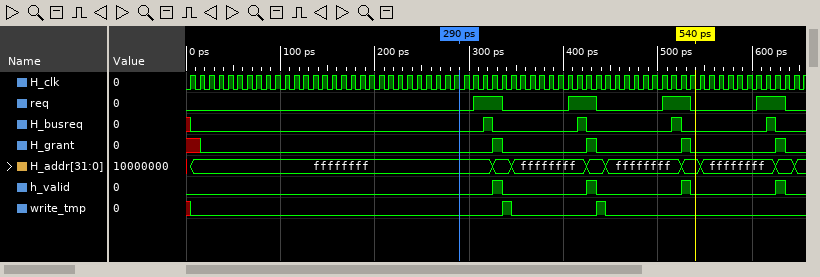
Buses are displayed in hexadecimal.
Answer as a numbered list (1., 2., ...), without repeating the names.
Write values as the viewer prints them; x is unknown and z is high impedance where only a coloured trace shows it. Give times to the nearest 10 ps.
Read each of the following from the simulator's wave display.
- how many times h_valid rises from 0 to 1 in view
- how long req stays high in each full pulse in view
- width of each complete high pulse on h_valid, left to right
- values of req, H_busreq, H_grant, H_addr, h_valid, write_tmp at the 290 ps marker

1. 4
2. 30 ps, 30 ps, 30 ps, 30 ps
3. 10 ps, 10 ps, 10 ps, 10 ps
4. req=0, H_busreq=0, H_grant=0, H_addr=ffffffff, h_valid=0, write_tmp=0
